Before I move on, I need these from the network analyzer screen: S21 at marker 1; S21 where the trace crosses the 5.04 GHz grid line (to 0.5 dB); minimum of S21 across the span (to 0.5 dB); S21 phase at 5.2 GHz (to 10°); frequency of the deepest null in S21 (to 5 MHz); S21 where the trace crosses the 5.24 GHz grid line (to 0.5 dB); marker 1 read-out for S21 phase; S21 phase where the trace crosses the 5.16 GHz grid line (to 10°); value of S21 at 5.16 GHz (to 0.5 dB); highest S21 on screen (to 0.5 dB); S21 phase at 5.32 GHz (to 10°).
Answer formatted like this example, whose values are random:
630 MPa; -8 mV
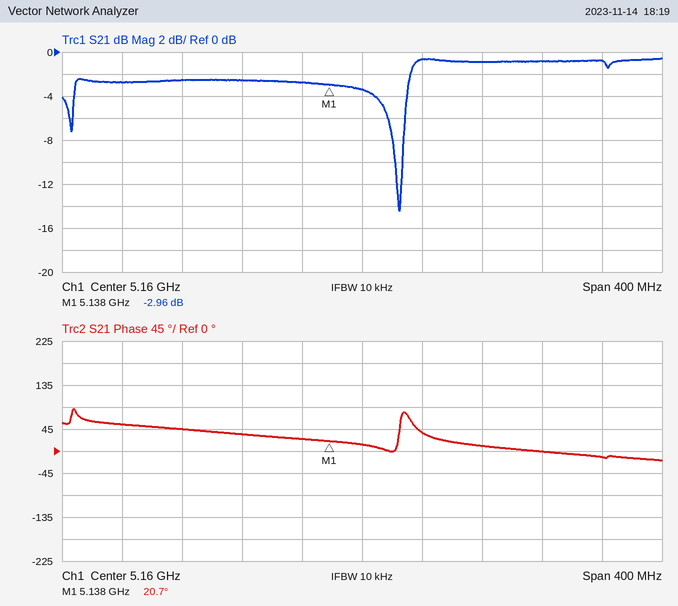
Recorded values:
-2.96 dB; -2.5 dB; -14.5 dB; 40°; 5.185 GHz; -1.0 dB; 20.7°; 10°; -3.5 dB; -0.5 dB; -10°
